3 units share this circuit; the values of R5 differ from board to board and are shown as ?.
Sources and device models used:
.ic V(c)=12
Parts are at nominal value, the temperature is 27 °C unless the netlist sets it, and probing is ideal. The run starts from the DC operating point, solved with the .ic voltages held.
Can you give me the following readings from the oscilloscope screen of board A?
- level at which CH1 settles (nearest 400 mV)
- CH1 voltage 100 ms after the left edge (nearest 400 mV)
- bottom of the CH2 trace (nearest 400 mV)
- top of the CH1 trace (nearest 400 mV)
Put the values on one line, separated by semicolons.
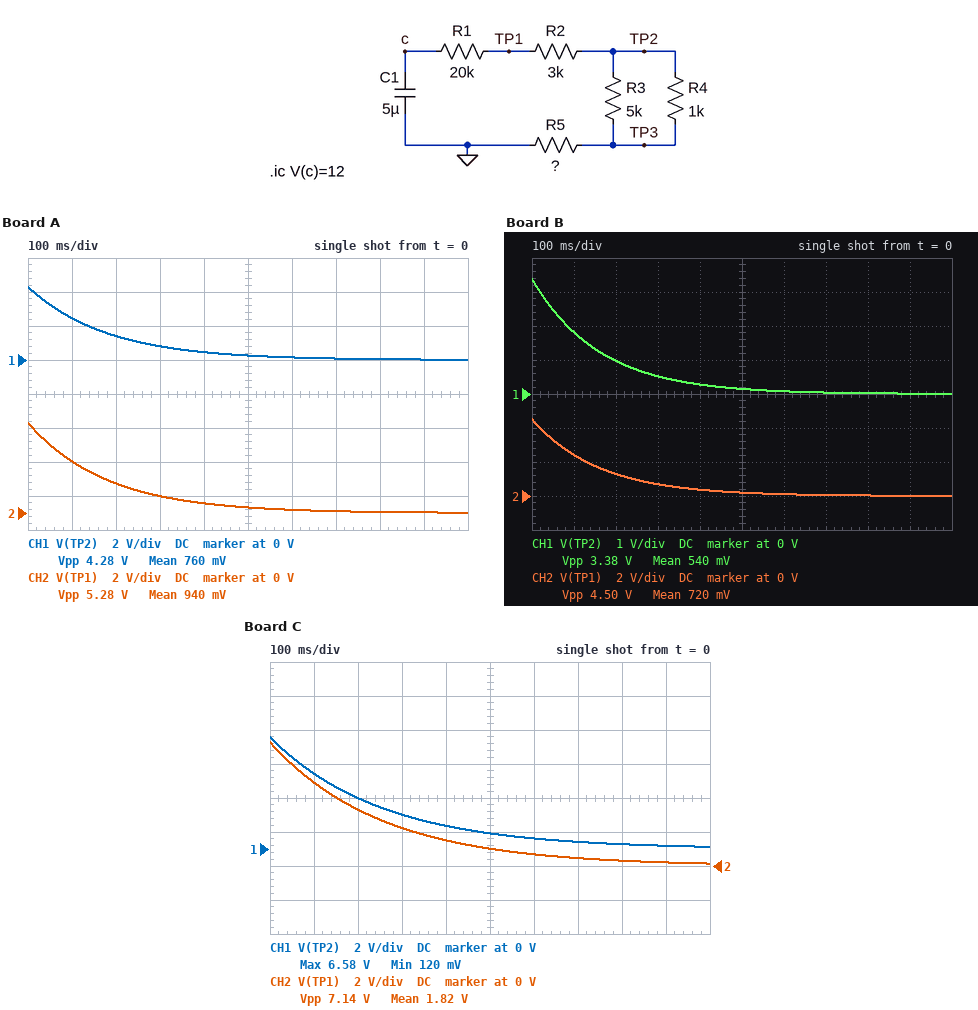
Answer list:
0 V; 2.4 V; 0 V; 4.4 V
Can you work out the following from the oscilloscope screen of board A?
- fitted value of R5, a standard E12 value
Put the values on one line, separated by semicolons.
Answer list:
12 kΩ
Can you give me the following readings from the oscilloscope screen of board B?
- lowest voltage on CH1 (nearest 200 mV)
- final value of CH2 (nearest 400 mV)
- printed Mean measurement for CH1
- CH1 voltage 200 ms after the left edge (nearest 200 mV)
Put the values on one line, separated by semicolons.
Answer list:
0 V; 0 V; 540 mV; 1.0 V
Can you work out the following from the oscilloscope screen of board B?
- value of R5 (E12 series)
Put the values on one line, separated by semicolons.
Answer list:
8.2 kΩ
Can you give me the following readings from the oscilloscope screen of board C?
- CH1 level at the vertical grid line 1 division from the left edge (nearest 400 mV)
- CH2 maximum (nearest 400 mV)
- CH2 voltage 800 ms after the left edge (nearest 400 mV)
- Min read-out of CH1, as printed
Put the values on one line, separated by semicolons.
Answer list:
4.4 V; 7.2 V; 400 mV; 120 mV
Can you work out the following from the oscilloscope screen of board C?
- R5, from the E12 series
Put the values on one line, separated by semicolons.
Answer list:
27 kΩ
